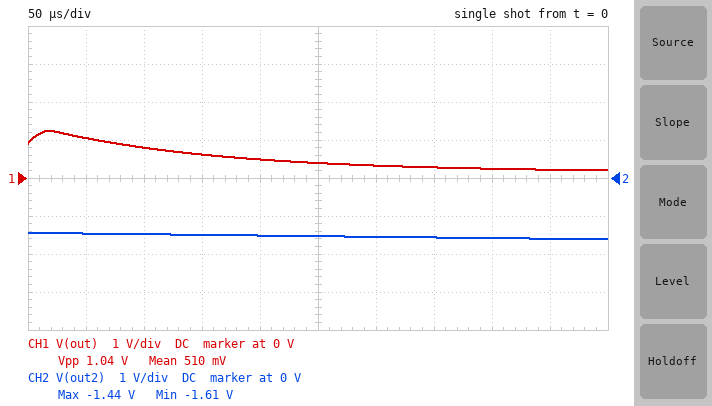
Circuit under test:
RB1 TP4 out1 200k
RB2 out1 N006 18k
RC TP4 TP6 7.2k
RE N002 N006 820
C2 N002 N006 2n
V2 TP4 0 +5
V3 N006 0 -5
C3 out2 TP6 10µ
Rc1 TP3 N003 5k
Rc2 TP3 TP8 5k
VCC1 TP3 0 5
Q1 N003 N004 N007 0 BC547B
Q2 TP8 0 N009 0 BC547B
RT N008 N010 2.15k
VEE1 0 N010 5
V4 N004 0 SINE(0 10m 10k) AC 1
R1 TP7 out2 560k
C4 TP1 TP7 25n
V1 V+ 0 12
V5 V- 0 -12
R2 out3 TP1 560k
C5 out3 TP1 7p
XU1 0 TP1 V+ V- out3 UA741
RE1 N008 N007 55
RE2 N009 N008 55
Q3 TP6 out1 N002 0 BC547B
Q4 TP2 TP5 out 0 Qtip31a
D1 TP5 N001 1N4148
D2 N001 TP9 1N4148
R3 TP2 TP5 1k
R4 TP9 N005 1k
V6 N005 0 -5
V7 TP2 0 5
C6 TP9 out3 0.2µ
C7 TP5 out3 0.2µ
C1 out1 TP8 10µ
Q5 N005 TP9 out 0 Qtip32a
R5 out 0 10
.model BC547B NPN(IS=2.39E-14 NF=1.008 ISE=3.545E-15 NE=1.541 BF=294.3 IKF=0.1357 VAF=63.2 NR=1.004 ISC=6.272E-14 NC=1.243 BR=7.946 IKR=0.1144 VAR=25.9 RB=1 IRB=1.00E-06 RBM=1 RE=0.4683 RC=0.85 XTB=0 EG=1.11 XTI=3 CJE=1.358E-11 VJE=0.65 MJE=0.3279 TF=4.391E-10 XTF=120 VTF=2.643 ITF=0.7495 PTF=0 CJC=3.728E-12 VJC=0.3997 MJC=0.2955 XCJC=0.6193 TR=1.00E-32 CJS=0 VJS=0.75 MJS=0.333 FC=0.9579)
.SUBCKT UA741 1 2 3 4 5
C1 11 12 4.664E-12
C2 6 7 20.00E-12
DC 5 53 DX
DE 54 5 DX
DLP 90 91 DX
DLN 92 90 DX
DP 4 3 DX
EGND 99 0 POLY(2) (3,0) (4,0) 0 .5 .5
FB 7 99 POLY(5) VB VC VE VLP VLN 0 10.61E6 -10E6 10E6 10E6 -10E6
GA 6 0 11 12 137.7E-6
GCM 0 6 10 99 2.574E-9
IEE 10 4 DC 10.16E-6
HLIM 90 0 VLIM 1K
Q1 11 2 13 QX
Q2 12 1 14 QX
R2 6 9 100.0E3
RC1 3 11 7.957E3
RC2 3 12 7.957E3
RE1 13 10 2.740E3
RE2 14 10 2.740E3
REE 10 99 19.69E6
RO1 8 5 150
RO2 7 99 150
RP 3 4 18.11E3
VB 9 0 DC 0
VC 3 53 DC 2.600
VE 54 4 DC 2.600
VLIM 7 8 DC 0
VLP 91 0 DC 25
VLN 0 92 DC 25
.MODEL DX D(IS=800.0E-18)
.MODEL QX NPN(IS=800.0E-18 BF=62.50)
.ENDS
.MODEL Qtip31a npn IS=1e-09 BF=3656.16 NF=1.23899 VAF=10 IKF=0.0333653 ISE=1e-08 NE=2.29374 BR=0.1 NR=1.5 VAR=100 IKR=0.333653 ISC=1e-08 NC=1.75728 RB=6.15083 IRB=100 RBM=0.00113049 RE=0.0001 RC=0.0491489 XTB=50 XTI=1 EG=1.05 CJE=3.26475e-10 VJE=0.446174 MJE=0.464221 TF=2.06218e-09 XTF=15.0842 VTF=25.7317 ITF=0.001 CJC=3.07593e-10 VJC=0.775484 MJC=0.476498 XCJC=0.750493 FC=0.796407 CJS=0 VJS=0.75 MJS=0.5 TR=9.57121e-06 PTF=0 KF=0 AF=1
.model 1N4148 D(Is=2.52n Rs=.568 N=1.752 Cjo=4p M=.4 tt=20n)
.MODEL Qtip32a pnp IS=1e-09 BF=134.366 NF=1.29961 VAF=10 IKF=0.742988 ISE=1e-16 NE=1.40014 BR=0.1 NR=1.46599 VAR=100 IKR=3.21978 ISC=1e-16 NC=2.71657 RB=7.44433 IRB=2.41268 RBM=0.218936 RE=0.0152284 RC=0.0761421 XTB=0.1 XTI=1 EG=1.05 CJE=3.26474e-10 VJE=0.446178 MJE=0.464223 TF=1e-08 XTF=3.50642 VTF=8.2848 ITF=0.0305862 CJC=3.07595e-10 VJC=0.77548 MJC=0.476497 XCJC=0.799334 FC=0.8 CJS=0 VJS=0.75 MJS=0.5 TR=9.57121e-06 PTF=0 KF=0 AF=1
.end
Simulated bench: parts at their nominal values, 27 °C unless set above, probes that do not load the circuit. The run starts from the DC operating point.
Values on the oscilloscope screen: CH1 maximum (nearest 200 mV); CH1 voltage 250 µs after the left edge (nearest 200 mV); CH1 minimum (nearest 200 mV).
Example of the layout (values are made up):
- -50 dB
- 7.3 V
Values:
- 1.2 V
- 400 mV
- 200 mV
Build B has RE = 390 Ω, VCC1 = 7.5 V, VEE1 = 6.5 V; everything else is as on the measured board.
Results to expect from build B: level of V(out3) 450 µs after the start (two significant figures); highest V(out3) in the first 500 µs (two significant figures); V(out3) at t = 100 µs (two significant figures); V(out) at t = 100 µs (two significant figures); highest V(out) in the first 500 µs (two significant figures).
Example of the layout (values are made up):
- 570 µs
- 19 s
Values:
- 1.8 V
- 1.9 V
- 1.6 V
- 860 mV
- 1.3 V
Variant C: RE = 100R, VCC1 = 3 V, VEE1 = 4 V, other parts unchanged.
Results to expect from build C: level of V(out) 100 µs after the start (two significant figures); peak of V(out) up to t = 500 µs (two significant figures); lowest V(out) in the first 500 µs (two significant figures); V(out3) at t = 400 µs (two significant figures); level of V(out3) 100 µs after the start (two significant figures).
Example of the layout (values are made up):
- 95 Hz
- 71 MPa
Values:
- 1.1 V
- 1.5 V
- 460 mV
- 2.7 V
- 2.0 V
